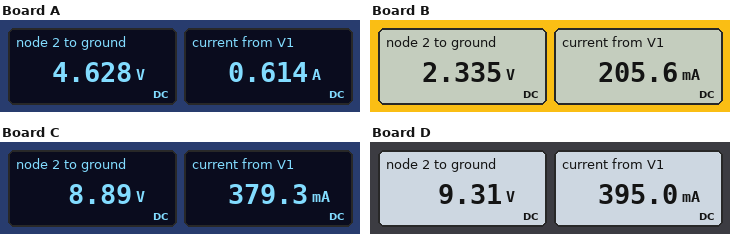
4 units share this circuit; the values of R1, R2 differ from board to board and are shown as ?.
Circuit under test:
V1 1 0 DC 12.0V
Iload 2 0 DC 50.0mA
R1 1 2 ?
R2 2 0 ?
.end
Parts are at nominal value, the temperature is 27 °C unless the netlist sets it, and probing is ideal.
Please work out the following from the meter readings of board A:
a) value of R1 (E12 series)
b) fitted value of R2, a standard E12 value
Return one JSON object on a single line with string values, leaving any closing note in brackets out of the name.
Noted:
{"value of R1": "12 Ω", "fitted value of R2, a standard E12 value": "8.2 Ω"}
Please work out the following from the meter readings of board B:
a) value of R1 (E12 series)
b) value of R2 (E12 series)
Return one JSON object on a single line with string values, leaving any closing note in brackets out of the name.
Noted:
{"value of R1": "47 Ω", "value of R2": "15 Ω"}
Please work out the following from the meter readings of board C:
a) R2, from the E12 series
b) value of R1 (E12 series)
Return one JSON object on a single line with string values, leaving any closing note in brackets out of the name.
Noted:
{"R2, from the E12 series": "27 Ω", "value of R1": "8.2 Ω"}
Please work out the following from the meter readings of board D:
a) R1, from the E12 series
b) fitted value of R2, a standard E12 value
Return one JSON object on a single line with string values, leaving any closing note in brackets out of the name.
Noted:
{"R1, from the E12 series": "6.8 Ω", "fitted value of R2, a standard E12 value": "27 Ω"}
